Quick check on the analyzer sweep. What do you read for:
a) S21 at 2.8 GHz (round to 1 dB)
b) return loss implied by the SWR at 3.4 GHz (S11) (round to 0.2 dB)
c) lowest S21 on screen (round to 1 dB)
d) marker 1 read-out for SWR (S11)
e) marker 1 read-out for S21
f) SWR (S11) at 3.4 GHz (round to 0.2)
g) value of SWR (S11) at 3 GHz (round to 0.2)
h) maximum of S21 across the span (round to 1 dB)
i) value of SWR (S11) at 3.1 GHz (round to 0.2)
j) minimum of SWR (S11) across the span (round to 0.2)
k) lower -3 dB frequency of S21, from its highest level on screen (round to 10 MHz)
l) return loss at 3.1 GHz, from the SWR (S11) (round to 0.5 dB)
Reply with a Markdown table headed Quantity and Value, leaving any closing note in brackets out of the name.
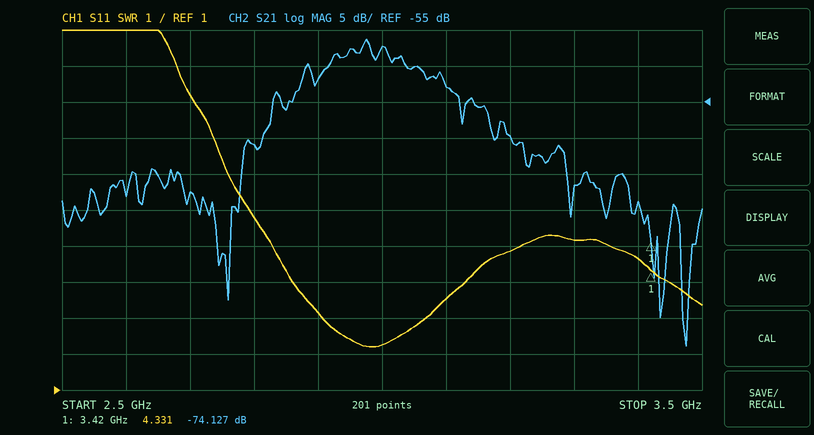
| Quantity | Value |
|---|---|
| S21 at 2.8 GHz | -61 dB |
| return loss implied by the SWR at 3.4 GHz (S11) | 3.8 dB |
| lowest S21 on screen | -89 dB |
| marker 1 read-out for SWR | 4.331 |
| marker 1 read-out for S21 | -74.127 dB |
| SWR (S11) at 3.4 GHz | 4.6 |
| value of SWR (S11) at 3 GHz | 2.2 |
| maximum of S21 across the span | -46 dB |
| value of SWR (S11) at 3.1 GHz | 3.6 |
| minimum of SWR (S11) across the span | 2.2 |
| lower -3 dB frequency of S21, from its highest level on screen | 2.92 GHz |
| return loss at 3.1 GHz, from the SWR (S11) | 5.0 dB |
